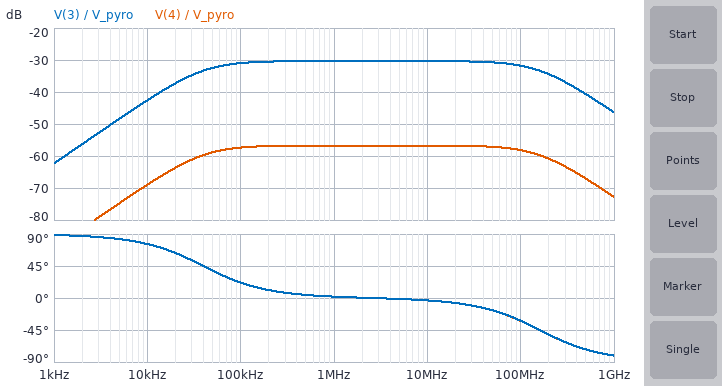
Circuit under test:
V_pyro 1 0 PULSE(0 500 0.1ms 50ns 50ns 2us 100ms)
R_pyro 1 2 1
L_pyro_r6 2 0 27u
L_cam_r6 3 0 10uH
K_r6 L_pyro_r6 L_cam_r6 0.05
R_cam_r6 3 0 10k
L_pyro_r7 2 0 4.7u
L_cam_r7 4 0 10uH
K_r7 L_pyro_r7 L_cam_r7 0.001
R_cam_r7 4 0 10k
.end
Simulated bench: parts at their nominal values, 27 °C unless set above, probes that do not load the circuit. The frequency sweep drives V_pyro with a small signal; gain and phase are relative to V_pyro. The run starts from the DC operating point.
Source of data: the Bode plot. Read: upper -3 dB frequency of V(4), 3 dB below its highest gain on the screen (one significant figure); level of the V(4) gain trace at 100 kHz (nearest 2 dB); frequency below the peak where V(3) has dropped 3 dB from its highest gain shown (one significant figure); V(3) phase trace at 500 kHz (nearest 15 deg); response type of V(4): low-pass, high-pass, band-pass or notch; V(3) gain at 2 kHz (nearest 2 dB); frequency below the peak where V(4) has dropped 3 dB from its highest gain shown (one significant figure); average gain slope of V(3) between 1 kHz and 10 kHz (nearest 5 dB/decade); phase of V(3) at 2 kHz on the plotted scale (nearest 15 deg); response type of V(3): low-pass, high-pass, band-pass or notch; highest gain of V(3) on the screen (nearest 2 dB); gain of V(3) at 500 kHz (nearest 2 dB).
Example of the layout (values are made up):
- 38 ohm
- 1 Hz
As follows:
- 200 MHz
- -58 dB
- 40 kHz
- 0 deg
- band-pass
- -56 dB
- 40 kHz
- 20 dB/decade
- 90 deg
- band-pass
- -30 dB
- -30 dB
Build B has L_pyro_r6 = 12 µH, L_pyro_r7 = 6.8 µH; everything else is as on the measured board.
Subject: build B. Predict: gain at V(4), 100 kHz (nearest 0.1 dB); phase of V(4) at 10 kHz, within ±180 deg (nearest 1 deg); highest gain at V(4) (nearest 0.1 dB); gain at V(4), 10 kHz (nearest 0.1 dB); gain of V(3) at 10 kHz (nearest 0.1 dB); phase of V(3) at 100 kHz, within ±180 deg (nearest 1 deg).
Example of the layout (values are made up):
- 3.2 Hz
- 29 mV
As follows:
- -58.9 dB
- 75 deg
- -58.3 dB
- -69.9 dB
- -38.4 dB
- 20 deg
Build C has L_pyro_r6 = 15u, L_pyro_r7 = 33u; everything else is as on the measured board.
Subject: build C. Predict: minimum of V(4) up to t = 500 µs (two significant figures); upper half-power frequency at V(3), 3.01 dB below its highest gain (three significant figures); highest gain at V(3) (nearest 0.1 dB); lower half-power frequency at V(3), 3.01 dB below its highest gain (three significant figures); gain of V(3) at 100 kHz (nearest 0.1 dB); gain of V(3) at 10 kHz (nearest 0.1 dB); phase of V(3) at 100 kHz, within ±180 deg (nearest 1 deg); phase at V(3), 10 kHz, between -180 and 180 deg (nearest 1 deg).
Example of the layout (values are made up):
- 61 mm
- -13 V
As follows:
- -50 mV
- 160 MHz
- -27.8 dB
- 15.4 kHz
- -27.9 dB
- -33.1 dB
- 9 deg
- 57 deg
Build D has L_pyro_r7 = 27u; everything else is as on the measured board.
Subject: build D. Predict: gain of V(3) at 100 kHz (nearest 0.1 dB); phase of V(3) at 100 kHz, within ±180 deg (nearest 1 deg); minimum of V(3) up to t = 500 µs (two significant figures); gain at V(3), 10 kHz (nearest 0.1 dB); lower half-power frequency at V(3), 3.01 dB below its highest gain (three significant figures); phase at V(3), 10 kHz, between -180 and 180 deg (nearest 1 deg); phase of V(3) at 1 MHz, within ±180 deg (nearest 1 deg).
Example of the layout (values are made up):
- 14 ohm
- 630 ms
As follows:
- -30.4 dB
- 7 deg
- -2.2 V
- -34.1 dB
- 11.8 kHz
- 50 deg
- 0 deg
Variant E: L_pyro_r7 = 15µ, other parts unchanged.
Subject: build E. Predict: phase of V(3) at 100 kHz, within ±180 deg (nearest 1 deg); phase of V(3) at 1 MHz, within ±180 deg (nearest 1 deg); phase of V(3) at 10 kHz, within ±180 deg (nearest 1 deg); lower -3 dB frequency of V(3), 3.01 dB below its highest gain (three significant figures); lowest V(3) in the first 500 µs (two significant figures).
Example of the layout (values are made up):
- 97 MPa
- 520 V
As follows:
- 9 deg
- 1 deg
- 59 deg
- 16.5 kHz
- -2.9 V
